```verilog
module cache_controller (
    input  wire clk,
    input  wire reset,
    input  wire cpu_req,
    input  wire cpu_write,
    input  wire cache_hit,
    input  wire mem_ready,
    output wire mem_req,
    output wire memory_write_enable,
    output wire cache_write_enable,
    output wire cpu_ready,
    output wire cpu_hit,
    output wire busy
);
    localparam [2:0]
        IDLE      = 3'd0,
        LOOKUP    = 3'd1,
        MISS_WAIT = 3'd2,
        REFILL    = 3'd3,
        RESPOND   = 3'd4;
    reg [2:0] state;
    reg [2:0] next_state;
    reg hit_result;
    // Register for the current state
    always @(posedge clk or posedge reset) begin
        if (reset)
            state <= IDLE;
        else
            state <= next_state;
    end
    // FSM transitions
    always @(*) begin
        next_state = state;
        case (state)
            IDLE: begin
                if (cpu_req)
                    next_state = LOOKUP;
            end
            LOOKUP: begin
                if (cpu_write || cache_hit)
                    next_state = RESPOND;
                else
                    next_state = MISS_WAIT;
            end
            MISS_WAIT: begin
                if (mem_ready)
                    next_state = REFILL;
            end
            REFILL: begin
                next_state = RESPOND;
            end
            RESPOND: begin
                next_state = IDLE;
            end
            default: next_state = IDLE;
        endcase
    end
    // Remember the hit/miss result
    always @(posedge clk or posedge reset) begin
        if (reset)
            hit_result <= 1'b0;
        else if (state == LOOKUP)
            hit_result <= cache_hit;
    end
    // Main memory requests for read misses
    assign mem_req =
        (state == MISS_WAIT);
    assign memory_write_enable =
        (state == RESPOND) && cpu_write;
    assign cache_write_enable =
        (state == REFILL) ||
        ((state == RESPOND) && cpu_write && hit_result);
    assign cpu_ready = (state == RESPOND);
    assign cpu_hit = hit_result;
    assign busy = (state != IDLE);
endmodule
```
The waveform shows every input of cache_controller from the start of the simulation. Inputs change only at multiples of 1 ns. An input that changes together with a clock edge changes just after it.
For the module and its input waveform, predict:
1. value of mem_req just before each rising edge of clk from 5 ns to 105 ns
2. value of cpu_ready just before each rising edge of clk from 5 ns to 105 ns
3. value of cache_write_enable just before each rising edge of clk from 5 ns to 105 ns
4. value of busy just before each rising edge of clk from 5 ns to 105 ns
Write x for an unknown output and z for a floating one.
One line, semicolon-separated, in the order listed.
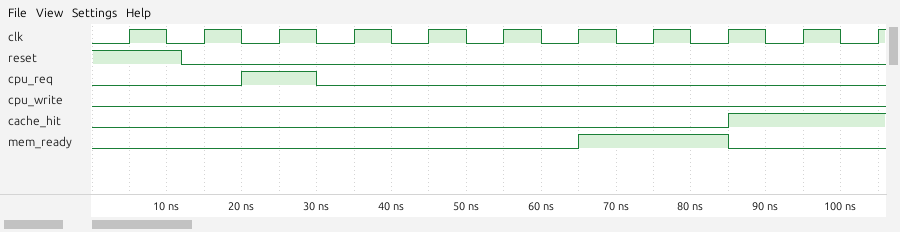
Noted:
0 0 0 0 1 1 1 1 0 0 0; 0 0 0 0 0 0 0 0 0 1 0; 0 0 0 0 0 0 0 0 1 0 0; 0 0 0 1 1 1 1 1 1 1 0
